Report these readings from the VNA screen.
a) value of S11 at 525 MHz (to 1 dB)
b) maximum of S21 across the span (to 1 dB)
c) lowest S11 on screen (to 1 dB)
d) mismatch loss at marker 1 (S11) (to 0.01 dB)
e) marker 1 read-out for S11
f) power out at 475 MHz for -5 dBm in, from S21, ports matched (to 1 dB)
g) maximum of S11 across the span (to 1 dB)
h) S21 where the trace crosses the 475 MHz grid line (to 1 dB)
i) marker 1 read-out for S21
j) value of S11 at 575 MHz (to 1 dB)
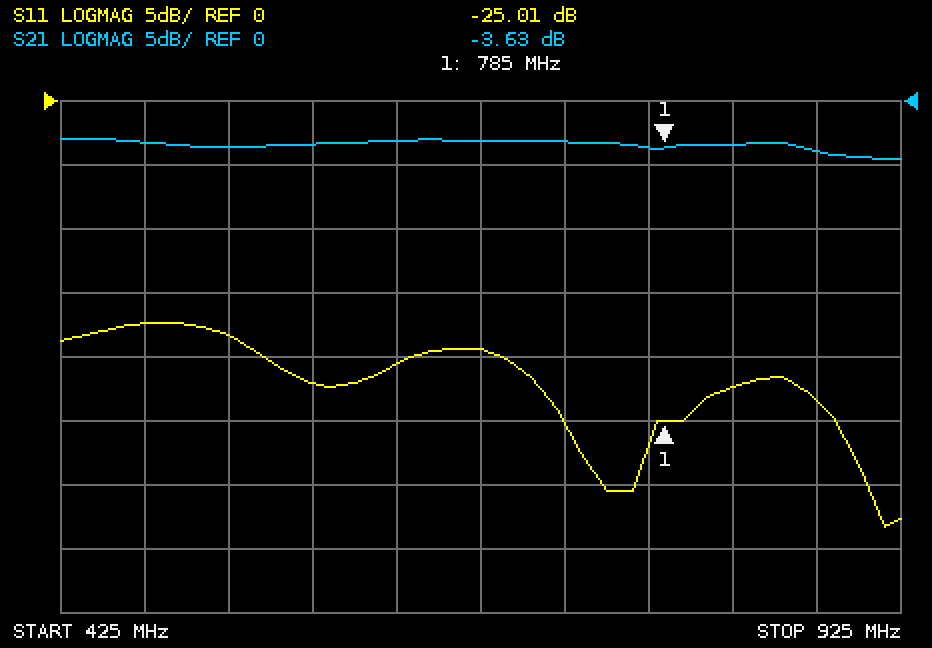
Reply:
-18 dB
-3 dB
-33 dB
0.01 dB
-25.01 dB
-8 dBm
-17 dB
-3 dB
-3.63 dB
-22 dB
